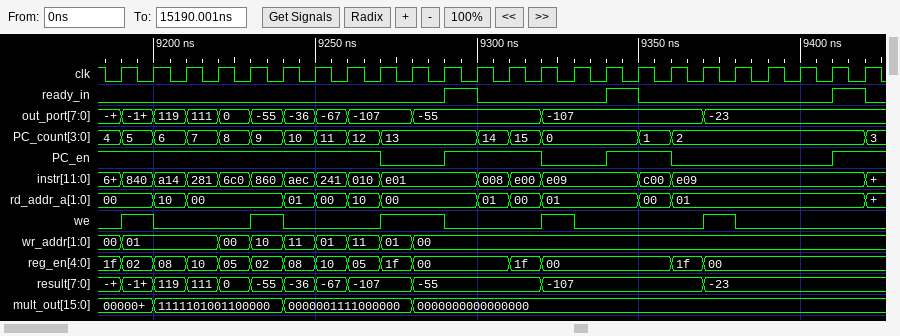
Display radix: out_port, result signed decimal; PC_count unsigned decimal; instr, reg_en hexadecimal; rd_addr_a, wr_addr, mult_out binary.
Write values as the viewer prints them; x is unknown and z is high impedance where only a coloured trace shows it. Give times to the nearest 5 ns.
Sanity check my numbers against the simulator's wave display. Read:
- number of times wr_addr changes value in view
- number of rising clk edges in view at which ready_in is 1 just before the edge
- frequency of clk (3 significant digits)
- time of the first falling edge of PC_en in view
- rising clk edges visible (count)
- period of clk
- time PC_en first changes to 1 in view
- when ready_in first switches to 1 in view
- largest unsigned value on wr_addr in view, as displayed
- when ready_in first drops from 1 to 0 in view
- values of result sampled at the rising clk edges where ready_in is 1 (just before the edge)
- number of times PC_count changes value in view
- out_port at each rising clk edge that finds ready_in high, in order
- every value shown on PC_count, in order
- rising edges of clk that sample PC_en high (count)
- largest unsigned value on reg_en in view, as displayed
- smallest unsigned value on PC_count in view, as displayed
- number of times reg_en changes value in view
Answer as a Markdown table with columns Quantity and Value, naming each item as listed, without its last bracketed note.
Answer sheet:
| Quantity | Value |
|---|---|
| number of times wr_addr changes value in view | 8 |
| number of rising clk edges in view at which ready_in is 1 just before the edge | 3 |
| frequency of clk | 100 MHz |
| time of the first falling edge of PC_en in view | 9270 ns |
| rising clk edges visible | 24 |
| period of clk | 10 ns |
| time PC_en first changes to 1 in view | 9290 ns |
| when ready_in first switches to 1 in view | 9290 ns |
| largest unsigned value on wr_addr in view, as displayed | 11 |
| when ready_in first drops from 1 to 0 in view | 9300 ns |
| values of result sampled at the rising clk edges where ready_in is 1 | -55, -107, -23 |
| number of times PC_count changes value in view | 15 |
| out_port at each rising clk edge that finds ready_in high, in order | -55, -107, -23 |
| every value shown on PC_count, in order | 4, 5, 6, 7, 8, 9, 10, 11, 12, 13, 14, 15, 0, 1, 2, 3 |
| rising edges of clk that sample PC_en high | 15 |
| largest unsigned value on reg_en in view, as displayed | 1f |
| smallest unsigned value on PC_count in view, as displayed | 0 |
| number of times reg_en changes value in view | 14 |
